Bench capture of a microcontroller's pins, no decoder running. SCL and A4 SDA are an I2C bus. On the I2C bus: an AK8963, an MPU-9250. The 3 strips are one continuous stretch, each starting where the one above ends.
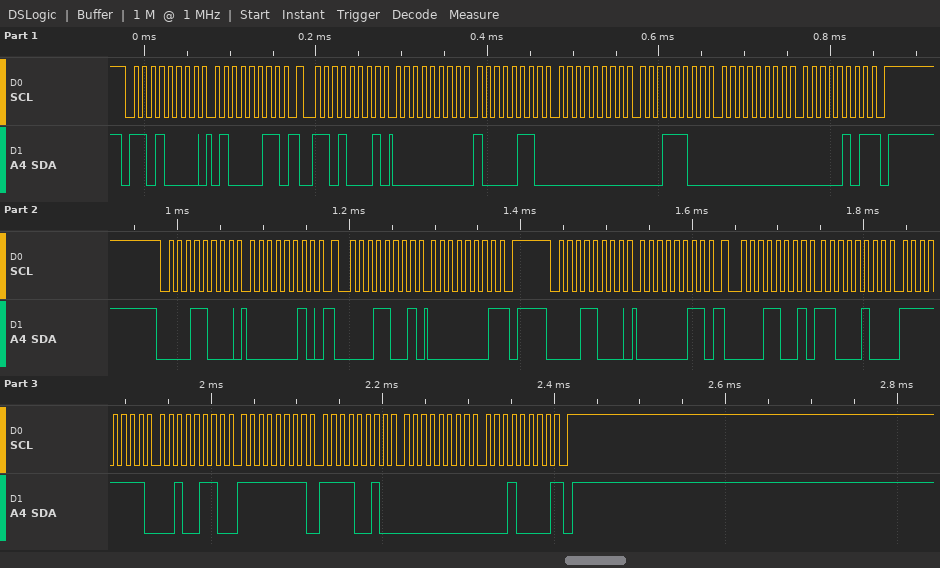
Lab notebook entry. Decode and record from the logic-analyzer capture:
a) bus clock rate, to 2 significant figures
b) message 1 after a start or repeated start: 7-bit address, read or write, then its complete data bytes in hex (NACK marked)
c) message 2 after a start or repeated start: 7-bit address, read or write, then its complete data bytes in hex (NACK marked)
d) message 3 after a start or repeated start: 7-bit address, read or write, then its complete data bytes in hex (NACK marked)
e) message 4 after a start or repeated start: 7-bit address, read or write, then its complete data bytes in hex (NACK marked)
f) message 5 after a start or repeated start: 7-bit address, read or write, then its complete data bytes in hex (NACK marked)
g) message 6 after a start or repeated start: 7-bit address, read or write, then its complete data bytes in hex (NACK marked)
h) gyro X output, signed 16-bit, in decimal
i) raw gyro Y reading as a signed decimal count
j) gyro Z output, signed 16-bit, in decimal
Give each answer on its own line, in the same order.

100 kHz
0x68 write: 43
0x68 read: 00 86 00 1C 00 05 NACK
0x0C write: 02
0x0C read: 01 NACK
0x0C write: 03
0x0C read: C4 FF 26 FF F2 00 10 NACK
134
28
5
